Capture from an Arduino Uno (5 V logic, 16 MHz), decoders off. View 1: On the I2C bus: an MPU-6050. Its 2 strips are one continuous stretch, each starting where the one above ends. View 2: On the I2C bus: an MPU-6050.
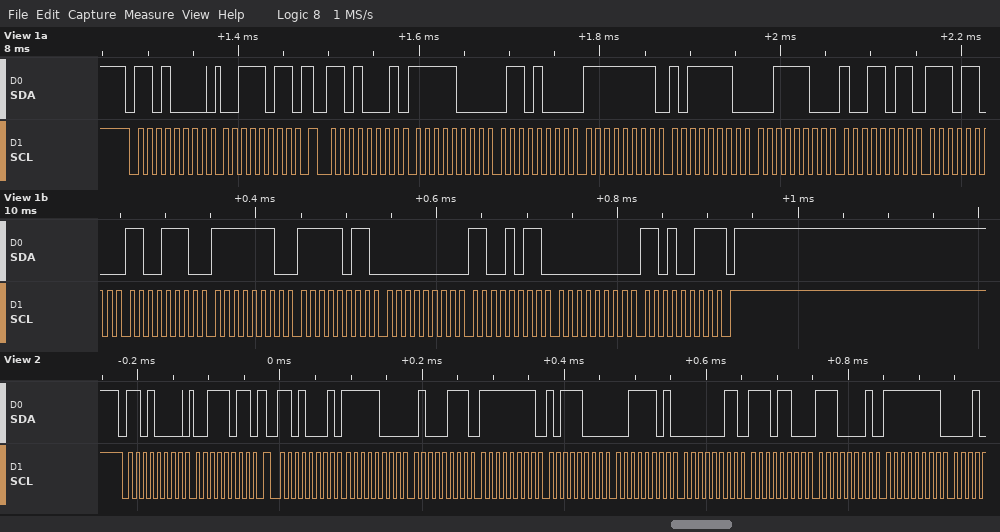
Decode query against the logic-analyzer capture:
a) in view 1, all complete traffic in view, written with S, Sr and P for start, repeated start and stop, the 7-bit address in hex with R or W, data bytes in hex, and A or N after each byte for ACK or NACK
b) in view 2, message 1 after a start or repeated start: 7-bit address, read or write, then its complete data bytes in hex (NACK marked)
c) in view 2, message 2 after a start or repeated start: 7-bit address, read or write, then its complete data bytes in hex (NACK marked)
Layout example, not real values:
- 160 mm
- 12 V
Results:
- S 68W A 3B A Sr 68R A F8 A 68 A FF A BE A 3C A 9B A EC A CE A FE A FB A 00 A CB A 00 A D3 N P
- 0x68 write: 3B
- 0x68 read: F8 47 FF B8 3D 03 EC E1 FF
